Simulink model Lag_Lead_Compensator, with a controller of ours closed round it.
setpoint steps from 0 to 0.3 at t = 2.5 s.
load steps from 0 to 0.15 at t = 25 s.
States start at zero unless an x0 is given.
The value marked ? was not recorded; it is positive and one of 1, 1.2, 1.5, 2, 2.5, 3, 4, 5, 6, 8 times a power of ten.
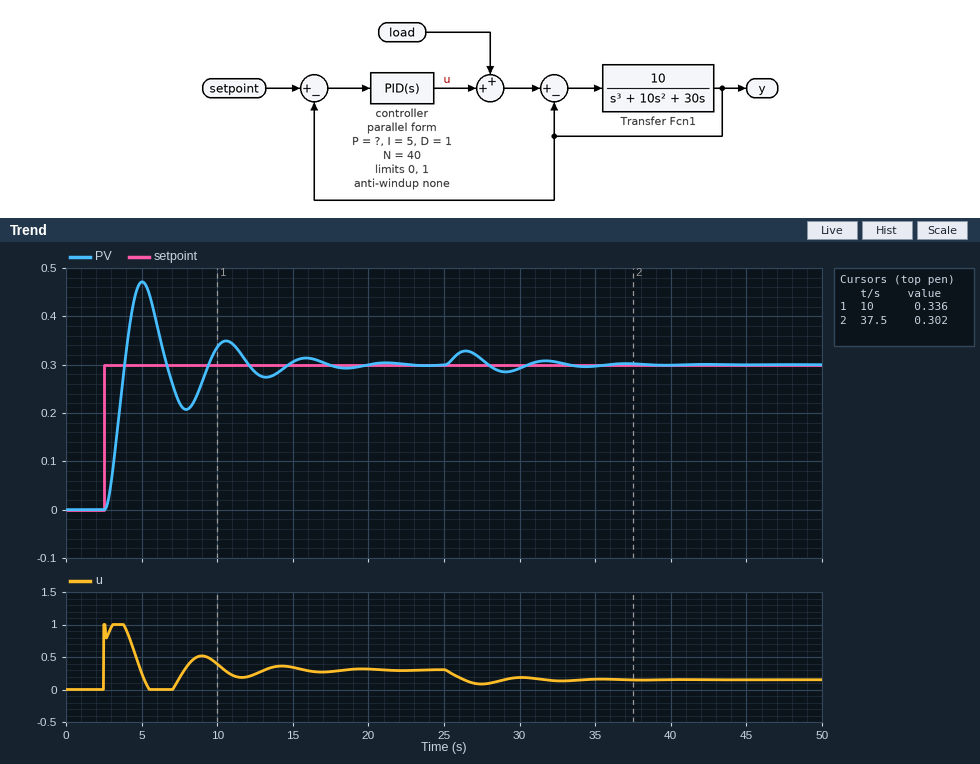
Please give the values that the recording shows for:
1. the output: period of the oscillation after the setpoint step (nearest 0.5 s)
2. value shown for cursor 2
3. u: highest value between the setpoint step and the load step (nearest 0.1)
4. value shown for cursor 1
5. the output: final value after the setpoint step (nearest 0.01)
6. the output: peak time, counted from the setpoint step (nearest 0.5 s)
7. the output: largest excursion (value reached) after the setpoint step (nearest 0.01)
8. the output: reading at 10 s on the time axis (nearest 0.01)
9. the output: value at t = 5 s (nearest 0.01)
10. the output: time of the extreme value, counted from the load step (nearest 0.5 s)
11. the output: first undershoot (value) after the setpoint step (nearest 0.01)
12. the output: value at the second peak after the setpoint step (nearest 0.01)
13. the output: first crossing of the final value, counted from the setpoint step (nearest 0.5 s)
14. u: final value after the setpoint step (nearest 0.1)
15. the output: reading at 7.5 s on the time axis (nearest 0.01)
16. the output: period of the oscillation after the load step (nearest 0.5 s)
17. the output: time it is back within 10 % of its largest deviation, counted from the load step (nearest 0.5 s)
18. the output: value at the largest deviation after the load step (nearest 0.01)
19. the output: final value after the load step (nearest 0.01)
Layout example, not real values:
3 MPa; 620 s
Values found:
5.5 s; 0.302; 1.0; 0.336; 0.30; 2.5 s; 0.47; 0.34; 0.47; 1.5 s; 0.21; 0.35; 1.5 s; 0.3; 0.22; 5.5 s; 10.0 s; 0.33; 0.30
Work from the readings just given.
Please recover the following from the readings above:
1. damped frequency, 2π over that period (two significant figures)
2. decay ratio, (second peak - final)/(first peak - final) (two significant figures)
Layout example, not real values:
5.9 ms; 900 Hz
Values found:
1.1 rad/s; 0.29
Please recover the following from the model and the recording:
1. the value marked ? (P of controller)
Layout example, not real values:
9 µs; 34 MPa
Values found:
2
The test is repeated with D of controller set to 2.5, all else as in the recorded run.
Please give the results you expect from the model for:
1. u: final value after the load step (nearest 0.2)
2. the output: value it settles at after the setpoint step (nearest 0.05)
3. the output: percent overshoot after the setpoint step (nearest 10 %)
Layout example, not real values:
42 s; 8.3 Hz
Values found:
0.2; 0.30; 50 %
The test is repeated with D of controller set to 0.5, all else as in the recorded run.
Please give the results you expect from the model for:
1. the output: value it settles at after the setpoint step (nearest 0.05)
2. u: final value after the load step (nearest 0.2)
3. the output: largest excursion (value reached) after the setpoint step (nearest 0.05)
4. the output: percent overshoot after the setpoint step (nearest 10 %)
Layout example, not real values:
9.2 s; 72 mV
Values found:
0.30; 0.2; 0.50; 60 %
